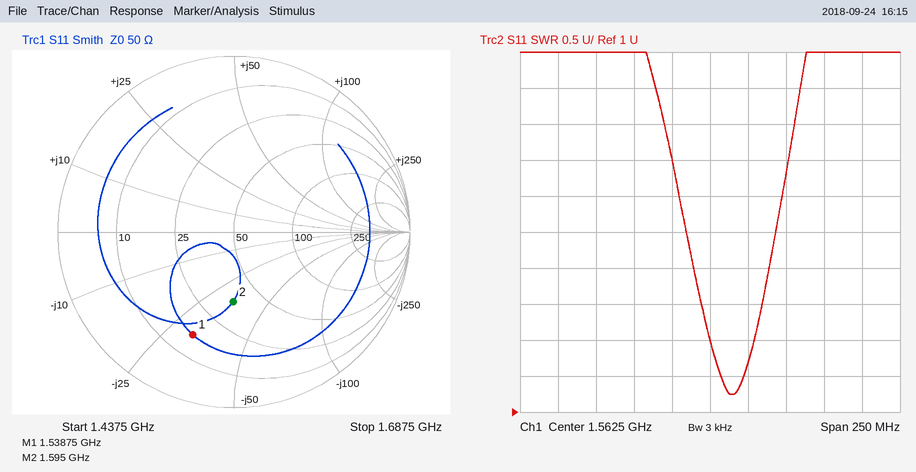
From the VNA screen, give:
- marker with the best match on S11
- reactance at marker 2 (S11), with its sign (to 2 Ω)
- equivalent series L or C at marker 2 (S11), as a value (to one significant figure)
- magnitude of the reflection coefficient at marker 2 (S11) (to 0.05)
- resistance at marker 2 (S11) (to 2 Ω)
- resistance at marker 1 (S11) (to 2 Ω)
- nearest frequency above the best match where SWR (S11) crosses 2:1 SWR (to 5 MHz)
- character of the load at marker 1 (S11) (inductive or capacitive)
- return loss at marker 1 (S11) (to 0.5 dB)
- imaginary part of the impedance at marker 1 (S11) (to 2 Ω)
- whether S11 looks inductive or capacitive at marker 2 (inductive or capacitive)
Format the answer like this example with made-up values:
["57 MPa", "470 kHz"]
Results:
["marker 2", "-34 Ω", "3 pF", "0.40", "36 Ω", "16 Ω", "1.590 GHz", "capacitive", "4.0 dB", "-32 Ω", "capacitive"]
